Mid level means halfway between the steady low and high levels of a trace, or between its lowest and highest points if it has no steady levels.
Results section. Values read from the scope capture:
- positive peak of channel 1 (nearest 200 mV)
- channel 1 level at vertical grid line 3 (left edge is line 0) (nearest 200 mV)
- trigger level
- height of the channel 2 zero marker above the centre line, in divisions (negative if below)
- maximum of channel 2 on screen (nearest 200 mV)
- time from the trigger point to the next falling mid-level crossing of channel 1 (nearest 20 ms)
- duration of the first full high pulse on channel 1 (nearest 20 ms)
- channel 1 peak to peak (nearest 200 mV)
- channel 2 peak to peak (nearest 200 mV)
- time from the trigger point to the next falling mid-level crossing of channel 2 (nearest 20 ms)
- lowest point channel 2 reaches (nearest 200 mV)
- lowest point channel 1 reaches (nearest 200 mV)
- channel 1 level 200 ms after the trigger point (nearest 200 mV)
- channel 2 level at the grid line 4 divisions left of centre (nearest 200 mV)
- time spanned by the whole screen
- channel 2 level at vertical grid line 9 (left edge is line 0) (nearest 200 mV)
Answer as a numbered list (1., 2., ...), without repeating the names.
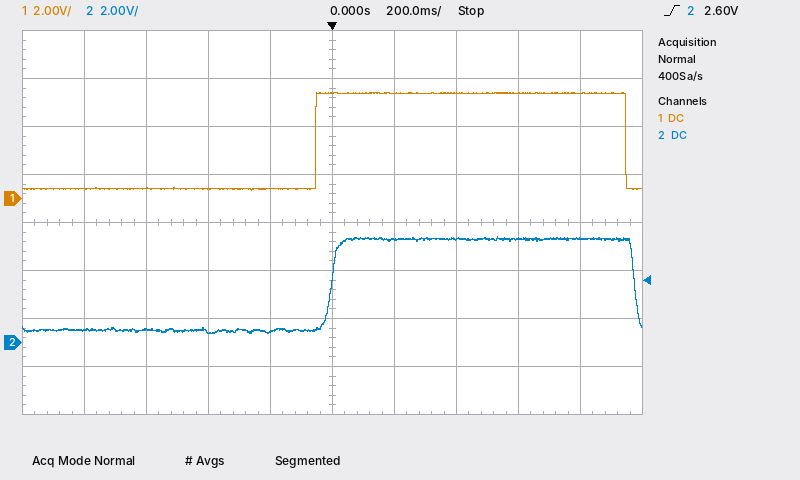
1. 4.4 V
2. 400 mV
3. 2.60 V
4. -2.5 div
5. 4.4 V
6. 940 ms
7. 1.00 s
8. 4.0 V
9. 4.0 V
10. 980 ms
11. 400 mV
12. 400 mV
13. 4.4 V
14. 600 mV
15. 2 s
16. 4.4 V
